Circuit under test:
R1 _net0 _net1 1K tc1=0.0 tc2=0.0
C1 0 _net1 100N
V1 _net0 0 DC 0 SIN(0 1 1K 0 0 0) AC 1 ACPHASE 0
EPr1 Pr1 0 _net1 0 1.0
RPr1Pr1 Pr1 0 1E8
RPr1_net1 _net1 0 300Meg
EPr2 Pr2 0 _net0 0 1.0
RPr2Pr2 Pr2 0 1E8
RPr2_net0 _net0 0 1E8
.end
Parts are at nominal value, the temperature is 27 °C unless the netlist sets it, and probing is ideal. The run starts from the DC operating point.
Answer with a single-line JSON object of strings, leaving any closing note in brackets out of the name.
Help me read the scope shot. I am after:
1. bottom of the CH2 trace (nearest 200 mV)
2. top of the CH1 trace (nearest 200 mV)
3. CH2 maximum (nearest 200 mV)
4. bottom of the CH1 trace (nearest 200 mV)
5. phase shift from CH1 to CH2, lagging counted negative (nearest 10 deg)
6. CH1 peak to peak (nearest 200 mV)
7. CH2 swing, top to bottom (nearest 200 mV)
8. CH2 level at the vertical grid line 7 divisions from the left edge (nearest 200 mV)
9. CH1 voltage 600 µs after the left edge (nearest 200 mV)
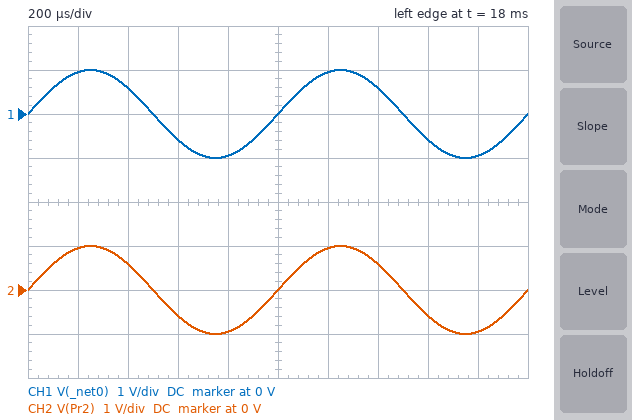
{"bottom of the CH2 trace": "-1.0 V", "top of the CH1 trace": "1.0 V", "CH2 maximum": "1.0 V", "bottom of the CH1 trace": "-1.0 V", "phase shift from CH1 to CH2, lagging counted negative": "0 deg", "CH1 peak to peak": "2.0 V", "CH2 swing, top to bottom": "2.0 V", "CH2 level at the vertical grid line 7 divisions from the left edge": "600 mV", "CH1 voltage 600 µs after the left edge": "-600 mV"}
